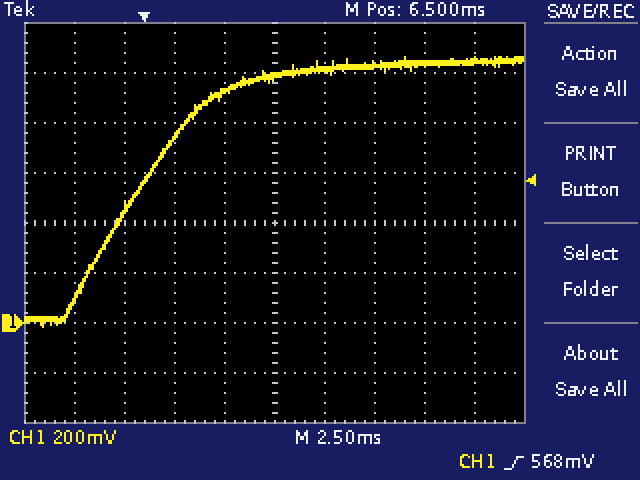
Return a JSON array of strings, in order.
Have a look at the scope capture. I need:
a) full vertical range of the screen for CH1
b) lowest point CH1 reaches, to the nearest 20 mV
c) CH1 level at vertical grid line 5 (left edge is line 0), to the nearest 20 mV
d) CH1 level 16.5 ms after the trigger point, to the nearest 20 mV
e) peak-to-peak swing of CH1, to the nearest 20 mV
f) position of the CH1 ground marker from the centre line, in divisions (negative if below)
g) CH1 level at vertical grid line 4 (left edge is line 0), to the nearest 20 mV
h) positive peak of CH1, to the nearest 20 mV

["1.6 V", "-20 mV", "980 mV", "1.04 V", "1.08 V", "-2.0 div", "920 mV", "1.06 V"]
